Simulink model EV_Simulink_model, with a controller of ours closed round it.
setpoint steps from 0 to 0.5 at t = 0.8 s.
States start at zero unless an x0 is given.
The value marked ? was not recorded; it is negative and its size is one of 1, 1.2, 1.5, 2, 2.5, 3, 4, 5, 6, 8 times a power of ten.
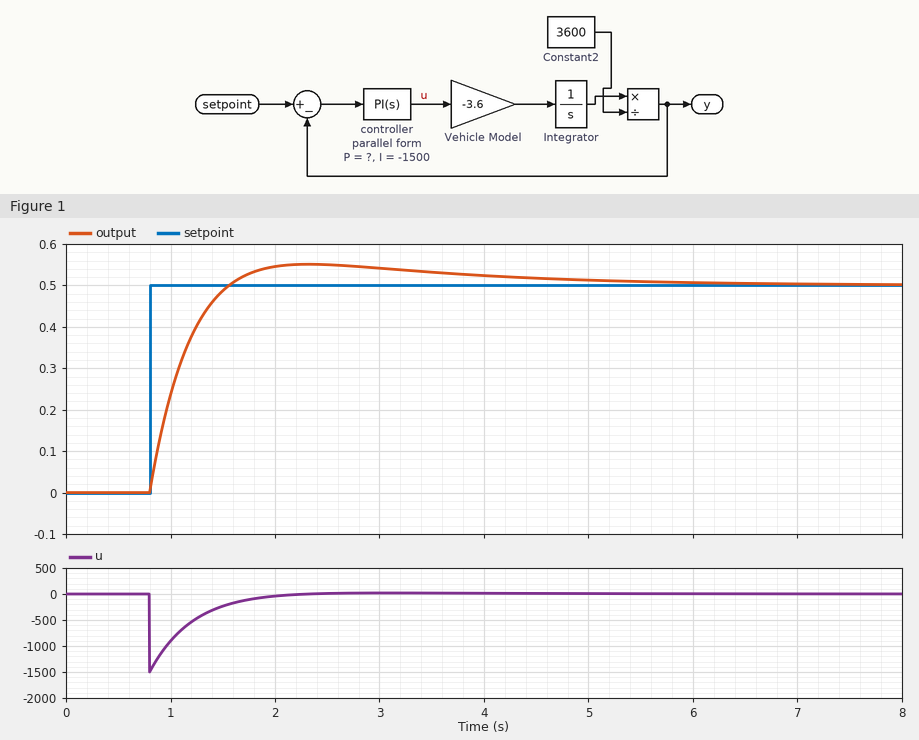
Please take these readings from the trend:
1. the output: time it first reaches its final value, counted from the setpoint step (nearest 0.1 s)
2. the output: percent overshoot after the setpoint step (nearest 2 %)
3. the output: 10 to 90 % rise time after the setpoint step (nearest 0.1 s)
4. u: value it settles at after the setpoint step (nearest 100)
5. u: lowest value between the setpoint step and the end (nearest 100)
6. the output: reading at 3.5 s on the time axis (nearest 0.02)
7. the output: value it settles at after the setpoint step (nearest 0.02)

0.8 s
10 %
0.5 s
0
-1500
0.54
0.50
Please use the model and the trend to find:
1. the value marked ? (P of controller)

-3000
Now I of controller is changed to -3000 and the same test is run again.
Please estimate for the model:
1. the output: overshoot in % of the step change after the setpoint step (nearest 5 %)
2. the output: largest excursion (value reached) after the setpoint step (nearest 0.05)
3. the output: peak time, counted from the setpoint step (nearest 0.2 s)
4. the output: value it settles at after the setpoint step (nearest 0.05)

15 %
0.60
1.2 s
0.50
